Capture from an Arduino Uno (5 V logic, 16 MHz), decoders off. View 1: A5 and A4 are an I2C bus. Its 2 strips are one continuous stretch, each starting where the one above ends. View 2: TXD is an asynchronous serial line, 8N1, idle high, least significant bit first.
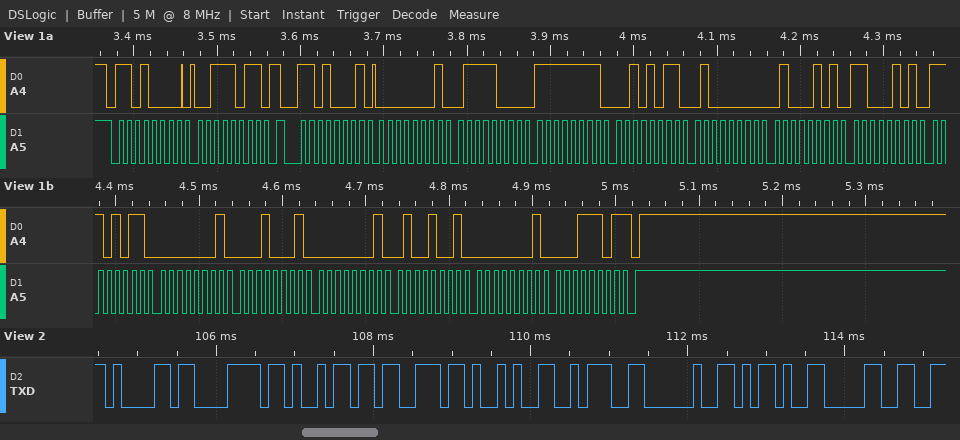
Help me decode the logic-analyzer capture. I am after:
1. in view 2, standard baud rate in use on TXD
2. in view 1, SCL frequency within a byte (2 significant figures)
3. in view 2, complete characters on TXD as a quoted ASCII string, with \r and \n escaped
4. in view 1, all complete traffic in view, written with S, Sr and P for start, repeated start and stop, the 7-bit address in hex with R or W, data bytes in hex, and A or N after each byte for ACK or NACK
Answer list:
9600 baud
100 kHz
"axis): -0"
S 68W A 3B A Sr 68R A 01 A 78 A FF A 2B A 40 A 45 A C5 A EB A 01 A 11 A 01 A 49 A 01 A 1D N P
